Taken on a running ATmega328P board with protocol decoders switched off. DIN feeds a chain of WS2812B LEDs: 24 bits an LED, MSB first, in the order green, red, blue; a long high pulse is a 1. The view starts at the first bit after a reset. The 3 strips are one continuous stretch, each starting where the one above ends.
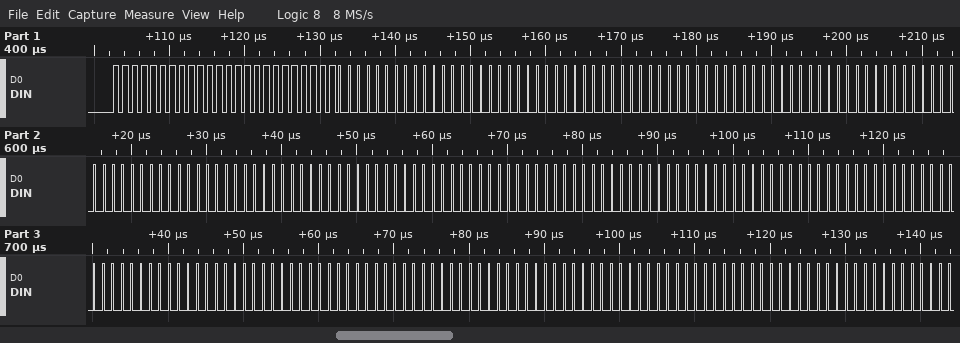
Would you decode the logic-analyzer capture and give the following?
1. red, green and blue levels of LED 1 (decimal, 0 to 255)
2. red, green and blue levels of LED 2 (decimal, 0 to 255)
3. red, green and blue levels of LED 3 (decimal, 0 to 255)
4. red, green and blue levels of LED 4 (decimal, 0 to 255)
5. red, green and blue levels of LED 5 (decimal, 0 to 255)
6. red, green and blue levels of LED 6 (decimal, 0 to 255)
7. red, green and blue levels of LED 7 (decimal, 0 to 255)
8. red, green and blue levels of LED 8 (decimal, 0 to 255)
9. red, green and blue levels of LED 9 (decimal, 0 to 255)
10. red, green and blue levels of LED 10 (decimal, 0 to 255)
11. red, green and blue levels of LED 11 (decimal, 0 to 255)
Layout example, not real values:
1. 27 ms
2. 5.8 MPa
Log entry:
1. 255, 255, 255
2. 0, 0, 0
3. 0, 0, 0
4. 0, 0, 0
5. 0, 0, 0
6. 0, 0, 0
7. 0, 0, 0
8. 0, 0, 0
9. 0, 0, 0
10. 0, 0, 0
11. 0, 0, 0
